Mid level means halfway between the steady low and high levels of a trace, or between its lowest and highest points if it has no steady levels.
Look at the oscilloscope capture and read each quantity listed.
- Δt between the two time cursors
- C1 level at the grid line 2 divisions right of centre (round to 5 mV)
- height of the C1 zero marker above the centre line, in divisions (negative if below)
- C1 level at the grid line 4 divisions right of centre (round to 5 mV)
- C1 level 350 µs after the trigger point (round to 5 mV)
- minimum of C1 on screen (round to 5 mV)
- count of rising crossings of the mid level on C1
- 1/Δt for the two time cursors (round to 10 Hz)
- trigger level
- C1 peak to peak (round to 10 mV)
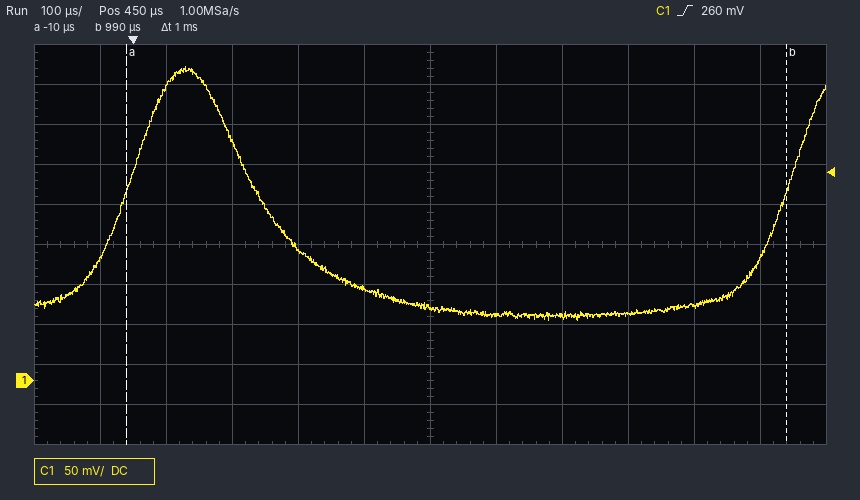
1 ms
80 mV
-3.4 div
95 mV
115 mV
75 mV
2
1.00 kHz
260 mV
320 mV
